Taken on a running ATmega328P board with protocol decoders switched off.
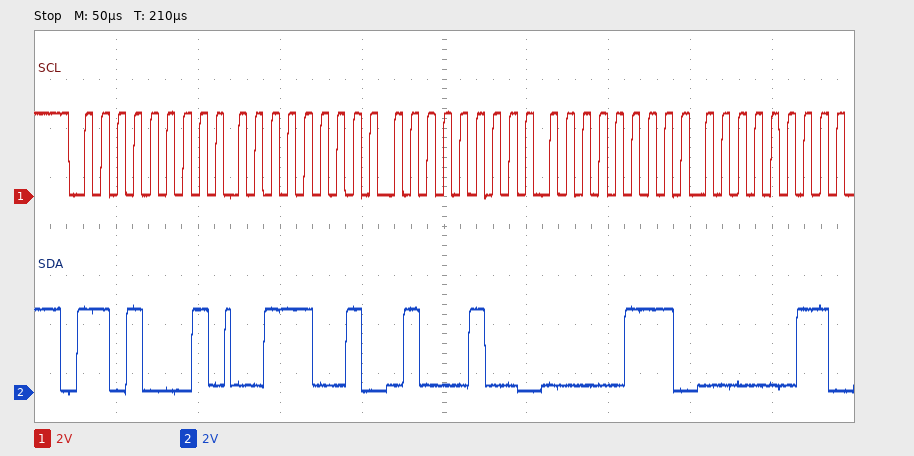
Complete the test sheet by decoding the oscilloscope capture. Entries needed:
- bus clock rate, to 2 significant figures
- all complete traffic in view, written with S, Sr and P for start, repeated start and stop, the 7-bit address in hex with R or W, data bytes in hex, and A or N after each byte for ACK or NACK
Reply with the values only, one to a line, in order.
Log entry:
100 kHz
S 68R A 39 A 44 A 07 A 03 A
